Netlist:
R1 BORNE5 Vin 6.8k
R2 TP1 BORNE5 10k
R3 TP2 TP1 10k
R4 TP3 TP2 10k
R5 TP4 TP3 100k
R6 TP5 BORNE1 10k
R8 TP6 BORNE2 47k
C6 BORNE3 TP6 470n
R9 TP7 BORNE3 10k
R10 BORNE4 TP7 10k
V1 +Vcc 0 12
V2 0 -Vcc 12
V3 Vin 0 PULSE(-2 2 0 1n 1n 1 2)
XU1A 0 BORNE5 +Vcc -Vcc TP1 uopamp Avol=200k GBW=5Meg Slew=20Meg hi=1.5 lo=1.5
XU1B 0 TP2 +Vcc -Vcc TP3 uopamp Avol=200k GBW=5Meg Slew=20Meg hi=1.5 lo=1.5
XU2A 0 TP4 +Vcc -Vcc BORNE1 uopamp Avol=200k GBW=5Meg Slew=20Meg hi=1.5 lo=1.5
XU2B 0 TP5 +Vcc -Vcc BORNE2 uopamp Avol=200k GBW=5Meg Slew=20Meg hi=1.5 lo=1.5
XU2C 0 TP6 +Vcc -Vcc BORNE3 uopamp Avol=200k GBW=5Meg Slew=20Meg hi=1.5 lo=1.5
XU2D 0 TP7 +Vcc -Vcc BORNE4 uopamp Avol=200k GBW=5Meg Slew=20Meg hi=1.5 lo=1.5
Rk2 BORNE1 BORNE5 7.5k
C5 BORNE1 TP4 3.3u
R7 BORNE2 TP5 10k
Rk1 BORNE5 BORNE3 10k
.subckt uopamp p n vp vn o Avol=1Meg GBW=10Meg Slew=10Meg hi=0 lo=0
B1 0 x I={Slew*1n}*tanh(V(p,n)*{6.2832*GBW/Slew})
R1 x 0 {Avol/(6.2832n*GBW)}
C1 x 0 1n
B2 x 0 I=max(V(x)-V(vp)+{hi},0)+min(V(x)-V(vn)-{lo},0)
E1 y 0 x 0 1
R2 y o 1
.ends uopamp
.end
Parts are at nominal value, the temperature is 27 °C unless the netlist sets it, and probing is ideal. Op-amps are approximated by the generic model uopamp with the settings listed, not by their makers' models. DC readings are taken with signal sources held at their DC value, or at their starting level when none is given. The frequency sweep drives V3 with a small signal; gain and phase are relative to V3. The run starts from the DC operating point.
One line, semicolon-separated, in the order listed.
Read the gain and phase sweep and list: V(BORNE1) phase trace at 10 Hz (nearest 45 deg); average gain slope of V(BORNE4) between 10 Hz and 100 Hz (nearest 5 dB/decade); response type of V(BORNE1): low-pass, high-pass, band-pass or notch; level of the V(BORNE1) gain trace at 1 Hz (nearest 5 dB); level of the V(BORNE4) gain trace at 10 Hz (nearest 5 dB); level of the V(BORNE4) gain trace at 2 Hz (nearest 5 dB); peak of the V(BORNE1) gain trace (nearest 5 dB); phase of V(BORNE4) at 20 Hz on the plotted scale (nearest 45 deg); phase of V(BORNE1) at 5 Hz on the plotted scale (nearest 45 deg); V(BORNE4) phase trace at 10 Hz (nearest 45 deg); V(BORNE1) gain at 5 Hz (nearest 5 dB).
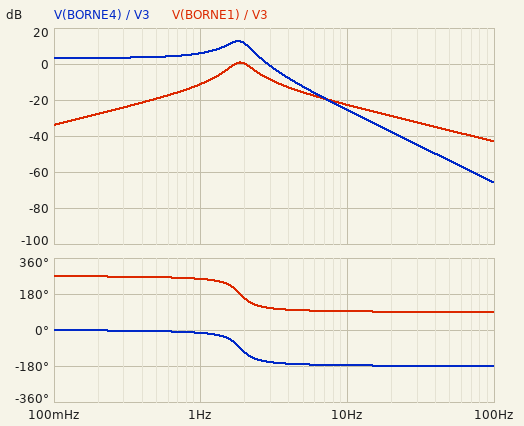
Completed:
90 deg; -40 dB/decade; band-pass; -10 dB; -25 dB; 10 dB; 0 dB; -180 deg; 90 deg; -180 deg; -15 dB
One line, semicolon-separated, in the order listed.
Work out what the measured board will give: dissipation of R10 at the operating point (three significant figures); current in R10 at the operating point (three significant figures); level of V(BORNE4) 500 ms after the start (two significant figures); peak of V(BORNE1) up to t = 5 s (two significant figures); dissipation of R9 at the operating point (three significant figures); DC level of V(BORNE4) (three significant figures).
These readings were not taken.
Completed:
865 µW; 294 µA; 1.3 V; 1.1 V; 865 µW; -2.94 V
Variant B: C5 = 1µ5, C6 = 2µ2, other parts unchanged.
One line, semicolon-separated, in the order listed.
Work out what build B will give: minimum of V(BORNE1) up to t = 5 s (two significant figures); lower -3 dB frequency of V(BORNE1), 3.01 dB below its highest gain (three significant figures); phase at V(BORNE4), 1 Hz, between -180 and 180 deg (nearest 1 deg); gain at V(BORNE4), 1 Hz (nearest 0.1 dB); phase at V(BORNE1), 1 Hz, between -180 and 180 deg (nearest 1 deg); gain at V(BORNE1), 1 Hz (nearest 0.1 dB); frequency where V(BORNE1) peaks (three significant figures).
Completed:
-2.5 V; 753 mHz; -66 deg; 3.8 dB; -156 deg; 0.1 dB; 1.28 Hz
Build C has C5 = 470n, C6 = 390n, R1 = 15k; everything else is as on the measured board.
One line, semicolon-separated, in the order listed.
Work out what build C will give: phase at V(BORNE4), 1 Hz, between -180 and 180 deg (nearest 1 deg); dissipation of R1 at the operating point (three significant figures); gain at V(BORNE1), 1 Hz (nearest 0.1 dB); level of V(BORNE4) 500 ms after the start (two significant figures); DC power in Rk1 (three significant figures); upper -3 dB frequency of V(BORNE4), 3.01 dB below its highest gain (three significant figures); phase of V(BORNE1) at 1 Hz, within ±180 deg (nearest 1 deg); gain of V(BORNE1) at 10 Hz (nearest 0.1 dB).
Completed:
-9 deg; 267 µW; -22.1 dB; 1.3 V; 178 µW; 6.44 Hz; -99 deg; -11.4 dB
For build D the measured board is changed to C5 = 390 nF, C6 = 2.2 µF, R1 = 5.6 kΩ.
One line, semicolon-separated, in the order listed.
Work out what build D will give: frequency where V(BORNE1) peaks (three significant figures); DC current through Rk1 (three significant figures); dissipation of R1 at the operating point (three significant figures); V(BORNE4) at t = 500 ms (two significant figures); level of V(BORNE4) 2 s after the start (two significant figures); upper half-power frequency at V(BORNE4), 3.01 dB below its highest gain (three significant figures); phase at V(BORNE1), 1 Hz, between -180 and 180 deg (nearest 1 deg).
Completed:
2.51 Hz; 357 µA; 714 µW; 3.5 V; -3.6 V; 1.44 Hz; -136 deg
